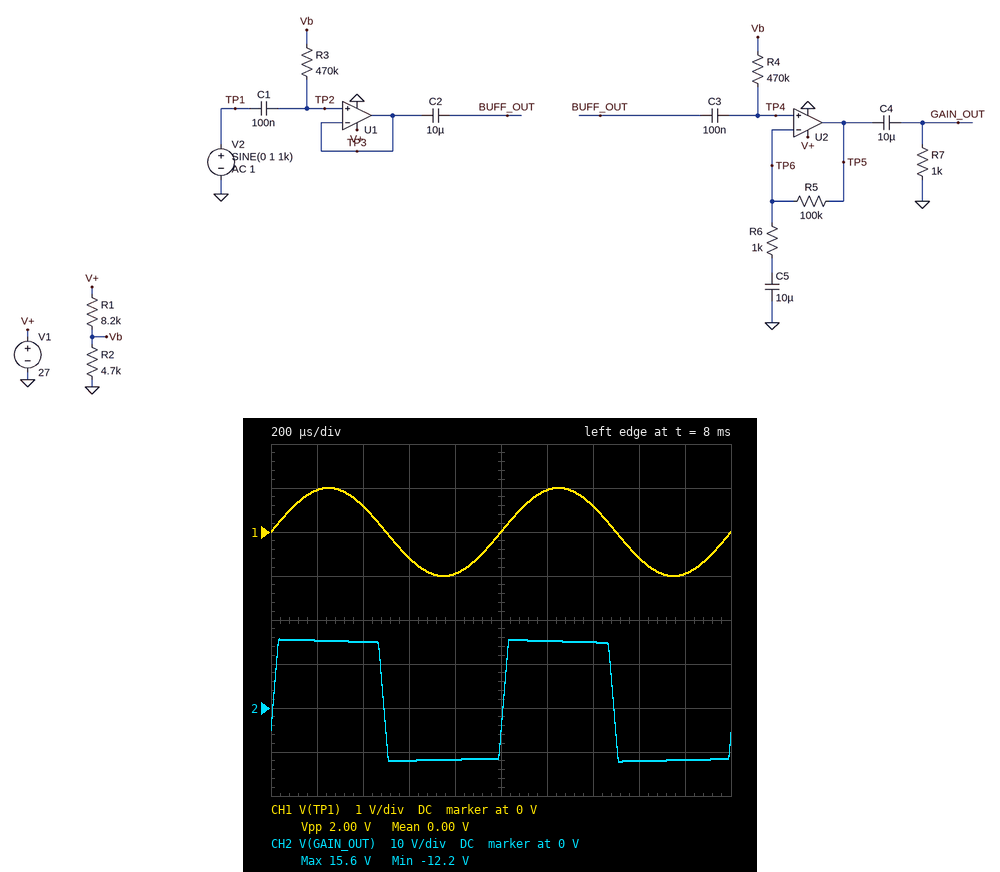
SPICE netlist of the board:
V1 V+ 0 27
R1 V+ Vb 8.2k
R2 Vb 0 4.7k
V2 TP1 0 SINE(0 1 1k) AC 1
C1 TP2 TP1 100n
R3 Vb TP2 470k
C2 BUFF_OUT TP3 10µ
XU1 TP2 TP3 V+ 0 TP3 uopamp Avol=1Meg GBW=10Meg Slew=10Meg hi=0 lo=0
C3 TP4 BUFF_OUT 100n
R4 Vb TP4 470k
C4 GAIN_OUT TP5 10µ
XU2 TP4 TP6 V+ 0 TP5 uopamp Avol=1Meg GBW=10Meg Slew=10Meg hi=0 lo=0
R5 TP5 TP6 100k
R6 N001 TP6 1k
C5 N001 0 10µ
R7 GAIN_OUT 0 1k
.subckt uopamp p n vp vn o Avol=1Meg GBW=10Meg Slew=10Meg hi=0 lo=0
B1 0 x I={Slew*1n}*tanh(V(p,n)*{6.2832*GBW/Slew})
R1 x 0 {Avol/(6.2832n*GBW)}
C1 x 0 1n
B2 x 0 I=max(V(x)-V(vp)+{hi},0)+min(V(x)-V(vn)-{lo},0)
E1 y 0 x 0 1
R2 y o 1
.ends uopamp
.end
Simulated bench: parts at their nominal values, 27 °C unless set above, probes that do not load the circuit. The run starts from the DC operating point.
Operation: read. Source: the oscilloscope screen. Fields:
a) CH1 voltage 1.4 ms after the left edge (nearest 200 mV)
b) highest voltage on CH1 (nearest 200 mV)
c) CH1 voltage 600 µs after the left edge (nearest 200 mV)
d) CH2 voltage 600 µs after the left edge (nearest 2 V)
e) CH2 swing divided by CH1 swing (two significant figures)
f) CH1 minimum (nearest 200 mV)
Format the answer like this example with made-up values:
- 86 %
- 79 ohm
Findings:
- 600 mV
- 1.0 V
- -600 mV
- -12 V
- 14
- -1.0 V
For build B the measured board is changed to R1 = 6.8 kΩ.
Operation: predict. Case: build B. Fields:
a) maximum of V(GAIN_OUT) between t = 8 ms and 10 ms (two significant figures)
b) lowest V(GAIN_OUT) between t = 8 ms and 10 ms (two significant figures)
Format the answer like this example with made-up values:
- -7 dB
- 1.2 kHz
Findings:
- 15 V
- -13 V
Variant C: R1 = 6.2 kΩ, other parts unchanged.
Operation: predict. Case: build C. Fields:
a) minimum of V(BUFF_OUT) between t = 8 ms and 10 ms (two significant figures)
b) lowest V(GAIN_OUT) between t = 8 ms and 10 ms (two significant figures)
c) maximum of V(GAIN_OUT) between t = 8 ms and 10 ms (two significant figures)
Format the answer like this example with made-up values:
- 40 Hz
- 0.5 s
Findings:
- -1.0 V
- -13 V
- 15 V
